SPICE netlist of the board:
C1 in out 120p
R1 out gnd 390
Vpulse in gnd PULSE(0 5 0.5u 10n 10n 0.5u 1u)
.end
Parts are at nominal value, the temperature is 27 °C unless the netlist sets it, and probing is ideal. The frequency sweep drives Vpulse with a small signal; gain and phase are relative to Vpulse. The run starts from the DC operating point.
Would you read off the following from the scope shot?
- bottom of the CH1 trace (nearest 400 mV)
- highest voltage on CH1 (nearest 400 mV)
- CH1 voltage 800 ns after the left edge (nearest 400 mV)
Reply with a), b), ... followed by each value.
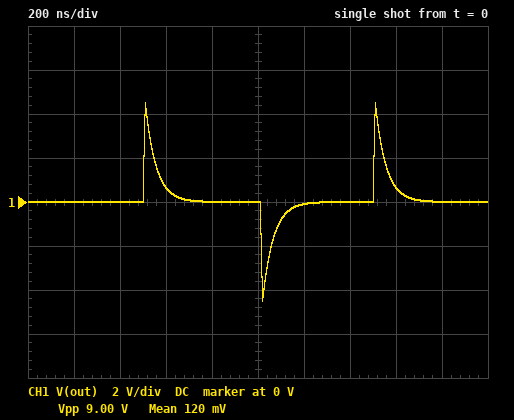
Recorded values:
a) -4.4 V
b) 4.4 V
c) 0 V
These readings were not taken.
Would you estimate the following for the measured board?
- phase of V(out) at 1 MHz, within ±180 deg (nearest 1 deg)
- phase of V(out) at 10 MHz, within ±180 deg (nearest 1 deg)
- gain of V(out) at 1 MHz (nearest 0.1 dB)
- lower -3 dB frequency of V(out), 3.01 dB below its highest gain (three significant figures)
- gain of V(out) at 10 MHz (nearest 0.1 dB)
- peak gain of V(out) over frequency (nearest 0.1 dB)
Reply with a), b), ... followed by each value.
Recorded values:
a) 74 deg
b) 19 deg
c) -11.0 dB
d) 3.40 MHz
e) -0.5 dB
f) 0 dB
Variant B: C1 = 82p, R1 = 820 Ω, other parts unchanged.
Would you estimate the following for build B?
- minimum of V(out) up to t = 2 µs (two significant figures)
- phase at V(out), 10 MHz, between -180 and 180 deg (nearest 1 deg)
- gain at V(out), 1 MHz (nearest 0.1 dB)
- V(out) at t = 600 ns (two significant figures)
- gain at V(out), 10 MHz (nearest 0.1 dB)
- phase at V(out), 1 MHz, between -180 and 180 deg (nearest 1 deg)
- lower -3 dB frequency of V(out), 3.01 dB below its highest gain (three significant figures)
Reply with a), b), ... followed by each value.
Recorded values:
a) -4.6 V
b) 13 deg
c) -8.2 dB
d) 1.2 V
e) -0.2 dB
f) 67 deg
g) 2.37 MHz
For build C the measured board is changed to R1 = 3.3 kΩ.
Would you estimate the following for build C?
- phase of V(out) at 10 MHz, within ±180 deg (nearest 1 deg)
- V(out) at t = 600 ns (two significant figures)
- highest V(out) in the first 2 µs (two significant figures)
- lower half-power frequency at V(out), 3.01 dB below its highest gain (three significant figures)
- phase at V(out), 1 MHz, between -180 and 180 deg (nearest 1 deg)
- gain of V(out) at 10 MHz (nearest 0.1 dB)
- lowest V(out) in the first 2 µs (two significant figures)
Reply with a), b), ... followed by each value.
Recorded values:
a) 2 deg
b) 3.9 V
c) 4.9 V
d) 402 kHz
e) 22 deg
f) 0 dB
g) -3.6 V
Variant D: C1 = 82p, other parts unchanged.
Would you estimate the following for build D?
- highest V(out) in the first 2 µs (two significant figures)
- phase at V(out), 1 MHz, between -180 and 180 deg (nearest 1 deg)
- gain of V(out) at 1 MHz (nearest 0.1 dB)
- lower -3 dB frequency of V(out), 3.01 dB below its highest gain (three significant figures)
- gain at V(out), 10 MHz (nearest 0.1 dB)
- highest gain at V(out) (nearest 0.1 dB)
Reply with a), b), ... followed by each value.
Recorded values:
a) 4.3 V
b) 79 deg
c) -14.1 dB
d) 4.98 MHz
e) -1.0 dB
f) 0 dB
